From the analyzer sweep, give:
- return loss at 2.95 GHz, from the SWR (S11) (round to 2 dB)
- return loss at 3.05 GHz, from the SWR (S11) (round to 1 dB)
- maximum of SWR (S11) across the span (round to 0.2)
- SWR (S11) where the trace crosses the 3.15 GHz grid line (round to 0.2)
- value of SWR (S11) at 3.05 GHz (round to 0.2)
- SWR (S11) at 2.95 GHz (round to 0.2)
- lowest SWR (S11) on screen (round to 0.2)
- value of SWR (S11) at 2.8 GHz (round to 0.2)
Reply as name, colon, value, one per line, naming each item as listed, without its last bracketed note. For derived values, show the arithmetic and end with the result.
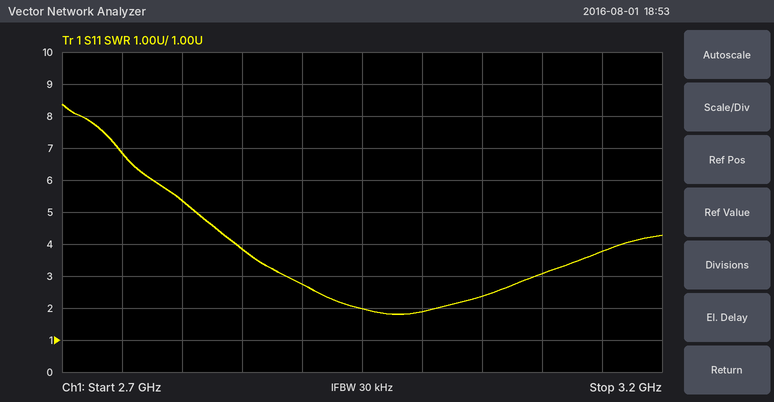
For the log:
return loss at 2.95 GHz, from the SWR (S11): −20 log10((2 − 1)/(2 + 1)) ≈ 10 dB
return loss at 3.05 GHz, from the SWR (S11): −20 log10((2.4 − 1)/(2.4 + 1)) ≈ 8 dB
maximum of SWR (S11) across the span: 8.4
SWR (S11) where the trace crosses the 3.15 GHz grid line: 3.8
value of SWR (S11) at 3.05 GHz: 2.4
SWR (S11) at 2.95 GHz: 2.0
lowest SWR (S11) on screen: 1.8
value of SWR (S11) at 2.8 GHz: 5.4
